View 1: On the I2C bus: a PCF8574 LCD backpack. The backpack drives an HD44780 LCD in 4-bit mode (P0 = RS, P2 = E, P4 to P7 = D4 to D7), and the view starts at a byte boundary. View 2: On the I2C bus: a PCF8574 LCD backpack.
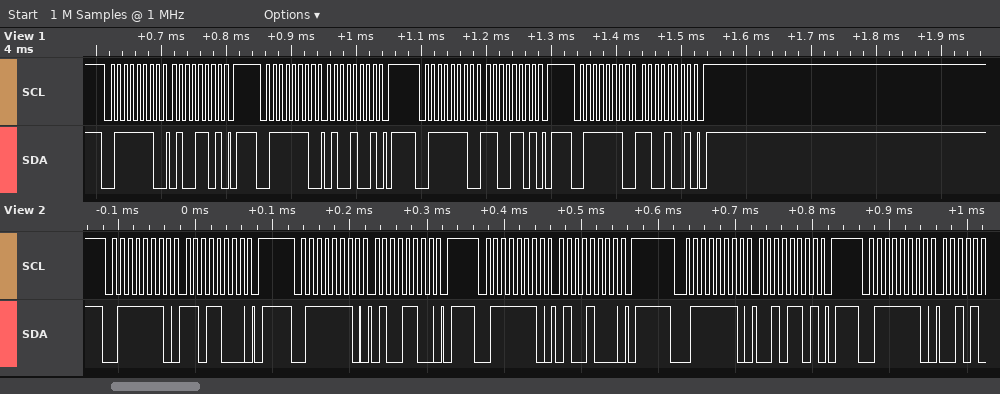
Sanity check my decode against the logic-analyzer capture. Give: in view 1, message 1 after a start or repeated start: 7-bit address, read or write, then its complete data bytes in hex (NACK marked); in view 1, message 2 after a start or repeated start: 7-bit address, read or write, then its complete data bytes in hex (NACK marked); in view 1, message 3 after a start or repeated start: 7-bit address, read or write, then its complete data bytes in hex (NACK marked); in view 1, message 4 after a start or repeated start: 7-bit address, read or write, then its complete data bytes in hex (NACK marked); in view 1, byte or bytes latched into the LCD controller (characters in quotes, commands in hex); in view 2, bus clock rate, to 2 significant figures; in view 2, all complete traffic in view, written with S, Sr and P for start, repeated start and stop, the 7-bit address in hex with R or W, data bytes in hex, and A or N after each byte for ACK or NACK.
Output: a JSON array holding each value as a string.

["0x3F write: 4D", "0x3F write: 49", "0x3F write: CD", "0x3F write: C9", "'L'", "100 kHz", "S 3FW A D8 A P S 3FW A 4C A P S 3FW A 48 A P S 3FW A 2D A P S 3FW A"]
